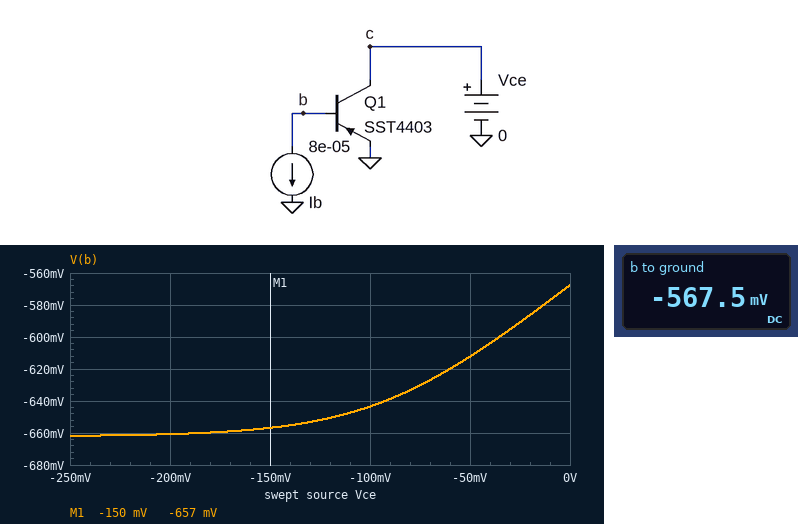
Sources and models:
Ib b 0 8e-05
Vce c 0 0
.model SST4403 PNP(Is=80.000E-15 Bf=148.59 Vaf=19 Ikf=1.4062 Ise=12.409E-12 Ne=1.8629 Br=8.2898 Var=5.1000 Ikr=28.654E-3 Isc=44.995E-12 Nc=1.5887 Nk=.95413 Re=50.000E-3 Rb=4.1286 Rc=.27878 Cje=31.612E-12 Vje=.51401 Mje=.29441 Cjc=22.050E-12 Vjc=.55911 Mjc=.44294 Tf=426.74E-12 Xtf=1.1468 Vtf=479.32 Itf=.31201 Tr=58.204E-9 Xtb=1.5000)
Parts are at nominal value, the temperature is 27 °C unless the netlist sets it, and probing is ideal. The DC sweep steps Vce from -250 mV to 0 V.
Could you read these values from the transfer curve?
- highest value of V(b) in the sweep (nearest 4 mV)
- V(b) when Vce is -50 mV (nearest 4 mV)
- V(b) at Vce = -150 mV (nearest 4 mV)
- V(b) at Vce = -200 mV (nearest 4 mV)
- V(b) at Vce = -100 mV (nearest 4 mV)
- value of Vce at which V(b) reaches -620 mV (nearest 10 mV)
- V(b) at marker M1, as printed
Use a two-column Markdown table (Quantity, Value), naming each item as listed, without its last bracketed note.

| Quantity | Value |
|---|---|
| highest value of V(b) in the sweep | -568 mV |
| V(b) when Vce is -50 mV | -612 mV |
| V(b) at Vce = -150 mV | -656 mV |
| V(b) at Vce = -200 mV | -660 mV |
| V(b) at Vce = -100 mV | -644 mV |
| value of Vce at which V(b) reaches -620 mV | -60 mV |
| V(b) at marker M1, as printed | -657 mV |
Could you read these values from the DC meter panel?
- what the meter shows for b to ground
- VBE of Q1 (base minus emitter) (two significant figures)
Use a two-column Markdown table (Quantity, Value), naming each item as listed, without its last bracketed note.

| Quantity | Value |
|---|---|
| what the meter shows for b to ground | -567.5 mV |
| VBE of Q1 (base minus emitter) | -570 mV |
